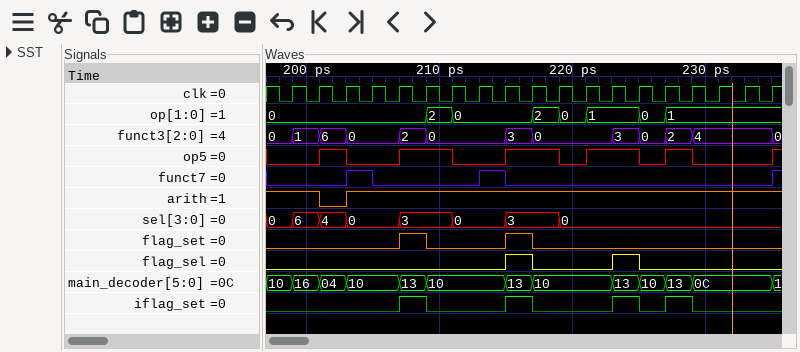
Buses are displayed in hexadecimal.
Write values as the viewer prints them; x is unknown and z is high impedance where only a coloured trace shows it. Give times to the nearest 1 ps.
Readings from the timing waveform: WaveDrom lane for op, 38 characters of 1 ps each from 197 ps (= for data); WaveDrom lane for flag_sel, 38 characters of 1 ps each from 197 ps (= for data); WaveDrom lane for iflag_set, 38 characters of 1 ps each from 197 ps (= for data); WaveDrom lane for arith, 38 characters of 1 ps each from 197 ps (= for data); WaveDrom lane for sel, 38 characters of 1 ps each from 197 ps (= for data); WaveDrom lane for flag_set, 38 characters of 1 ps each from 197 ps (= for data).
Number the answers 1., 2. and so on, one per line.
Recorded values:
1. {name: 'op', wave: '=...........=.=.....=.=.=...=.=.......', data: '0 2 0 2 0 1 0 1'}
2. {name: 'flag_sel', wave: '0.................1.0.....1.0.........'}
3. {name: 'iflag_set', wave: '0.........1.0.....1.0.....1.0.1.0.....'}
4. {name: 'arith', wave: '1...0.1...............................'}
5. {name: 'sel', wave: '=.=.=.=...=...=...=...=...............', data: '0 6 4 0 3 0 3 0'}
6. {name: 'flag_set', wave: '0.........1.0.....1.0.................'}
